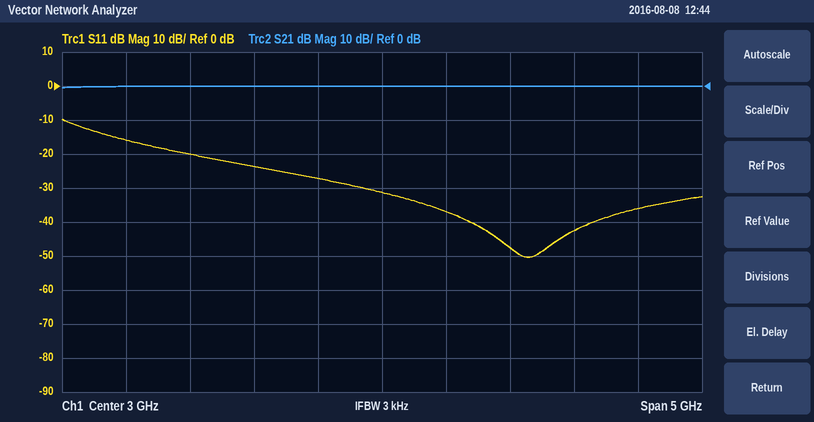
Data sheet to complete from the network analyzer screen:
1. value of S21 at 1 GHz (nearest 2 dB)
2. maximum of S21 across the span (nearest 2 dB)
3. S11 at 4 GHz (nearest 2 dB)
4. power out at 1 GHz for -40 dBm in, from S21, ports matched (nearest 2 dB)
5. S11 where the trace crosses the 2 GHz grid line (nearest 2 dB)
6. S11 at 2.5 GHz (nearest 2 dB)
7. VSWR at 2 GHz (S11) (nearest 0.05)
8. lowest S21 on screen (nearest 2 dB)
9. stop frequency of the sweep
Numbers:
0 dB
0 dB
-48 dB
-40 dBm
-24 dB
-28 dB
1.15
0 dB
5.5 GHz
